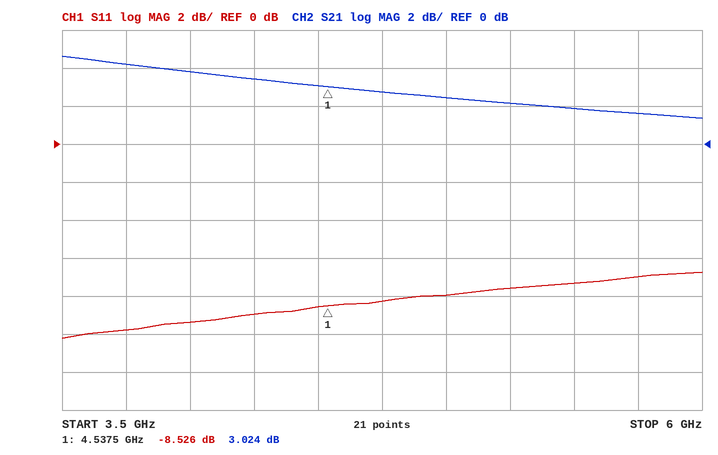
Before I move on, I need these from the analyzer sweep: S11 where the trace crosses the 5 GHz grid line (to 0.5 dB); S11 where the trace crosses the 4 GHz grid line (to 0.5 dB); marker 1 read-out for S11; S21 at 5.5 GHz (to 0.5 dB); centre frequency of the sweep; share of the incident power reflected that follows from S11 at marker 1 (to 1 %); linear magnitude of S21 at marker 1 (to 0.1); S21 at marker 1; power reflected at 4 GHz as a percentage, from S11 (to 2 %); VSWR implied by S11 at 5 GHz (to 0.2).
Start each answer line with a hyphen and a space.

- -8.0 dB
- -9.5 dB
- -8.526 dB
- 2.0 dB
- 4.75 GHz
- 14 %
- 1.4
- 3.024 dB
- 12 %
- 2.4
